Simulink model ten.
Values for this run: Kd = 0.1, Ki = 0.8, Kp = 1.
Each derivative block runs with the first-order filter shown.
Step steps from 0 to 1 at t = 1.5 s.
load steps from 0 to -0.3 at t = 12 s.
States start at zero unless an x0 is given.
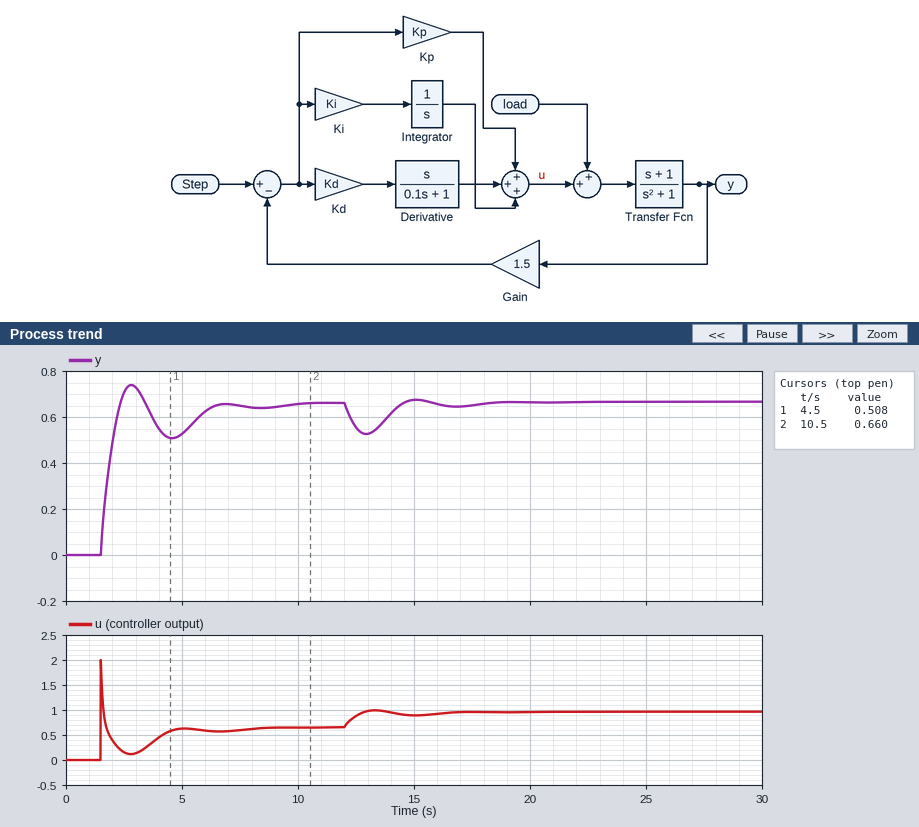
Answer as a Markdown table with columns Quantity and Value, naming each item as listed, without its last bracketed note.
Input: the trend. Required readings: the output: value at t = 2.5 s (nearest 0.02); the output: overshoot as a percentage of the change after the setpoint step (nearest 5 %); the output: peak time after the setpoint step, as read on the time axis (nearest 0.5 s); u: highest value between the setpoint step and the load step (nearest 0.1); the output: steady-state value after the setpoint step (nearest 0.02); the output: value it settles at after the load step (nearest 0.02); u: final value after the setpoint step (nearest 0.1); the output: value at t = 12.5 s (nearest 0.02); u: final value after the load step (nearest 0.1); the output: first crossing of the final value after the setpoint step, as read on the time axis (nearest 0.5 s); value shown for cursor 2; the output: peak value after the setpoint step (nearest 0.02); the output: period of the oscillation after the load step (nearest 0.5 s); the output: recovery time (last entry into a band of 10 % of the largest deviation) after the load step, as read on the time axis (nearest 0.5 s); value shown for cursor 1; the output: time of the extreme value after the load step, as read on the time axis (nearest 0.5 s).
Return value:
| Quantity | Value |
|---|---|
| the output: value at t = 2.5 s | 0.70 |
| the output: overshoot as a percentage of the change after the setpoint step | 10 % |
| the output: peak time after the setpoint step, as read on the time axis | 3.0 s |
| u: highest value between the setpoint step and the load step | 2.0 |
| the output: steady-state value after the setpoint step | 0.66 |
| the output: value it settles at after the load step | 0.66 |
| u: final value after the setpoint step | 0.7 |
| the output: value at t = 12.5 s | 0.56 |
| u: final value after the load step | 1.0 |
| the output: first crossing of the final value after the setpoint step, as read on the time axis | 2.5 s |
| value shown for cursor 2 | 0.660 |
| the output: peak value after the setpoint step | 0.74 |
| the output: period of the oscillation after the load step | 4.0 s |
| the output: recovery time (last entry into a band of 10 % of the largest deviation) after the load step, as read on the time axis | 17.5 s |
| value shown for cursor 1 | 0.508 |
| the output: time of the extreme value after the load step, as read on the time axis | 13.0 s |
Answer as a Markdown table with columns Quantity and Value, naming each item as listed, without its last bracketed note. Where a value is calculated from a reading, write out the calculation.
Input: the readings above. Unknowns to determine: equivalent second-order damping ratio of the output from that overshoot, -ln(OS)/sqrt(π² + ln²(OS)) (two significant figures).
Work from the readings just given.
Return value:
| Quantity | Value |
|---|---|
| equivalent second-order damping ratio of the output from that overshoot, -ln(OS)/sqrt(π² + ln²(OS)) | ln(0.1) = -2.303; 2.303 / sqrt(9.870 + 5.302) = 0.59 |
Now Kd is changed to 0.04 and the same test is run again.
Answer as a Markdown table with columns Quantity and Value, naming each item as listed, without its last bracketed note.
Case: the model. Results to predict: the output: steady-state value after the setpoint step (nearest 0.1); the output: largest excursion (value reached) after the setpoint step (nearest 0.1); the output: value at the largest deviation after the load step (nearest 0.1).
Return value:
| Quantity | Value |
|---|---|
| the output: steady-state value after the setpoint step | 0.7 |
| the output: largest excursion (value reached) after the setpoint step | 0.8 |
| the output: value at the largest deviation after the load step | 0.5 |
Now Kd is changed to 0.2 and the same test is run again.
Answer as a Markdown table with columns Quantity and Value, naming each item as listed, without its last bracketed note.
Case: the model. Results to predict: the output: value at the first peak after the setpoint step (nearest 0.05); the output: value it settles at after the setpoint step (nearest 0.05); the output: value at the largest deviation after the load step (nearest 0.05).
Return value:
| Quantity | Value |
|---|---|
| the output: value at the first peak after the setpoint step | 0.70 |
| the output: value it settles at after the setpoint step | 0.65 |
| the output: value at the largest deviation after the load step | 0.55 |
